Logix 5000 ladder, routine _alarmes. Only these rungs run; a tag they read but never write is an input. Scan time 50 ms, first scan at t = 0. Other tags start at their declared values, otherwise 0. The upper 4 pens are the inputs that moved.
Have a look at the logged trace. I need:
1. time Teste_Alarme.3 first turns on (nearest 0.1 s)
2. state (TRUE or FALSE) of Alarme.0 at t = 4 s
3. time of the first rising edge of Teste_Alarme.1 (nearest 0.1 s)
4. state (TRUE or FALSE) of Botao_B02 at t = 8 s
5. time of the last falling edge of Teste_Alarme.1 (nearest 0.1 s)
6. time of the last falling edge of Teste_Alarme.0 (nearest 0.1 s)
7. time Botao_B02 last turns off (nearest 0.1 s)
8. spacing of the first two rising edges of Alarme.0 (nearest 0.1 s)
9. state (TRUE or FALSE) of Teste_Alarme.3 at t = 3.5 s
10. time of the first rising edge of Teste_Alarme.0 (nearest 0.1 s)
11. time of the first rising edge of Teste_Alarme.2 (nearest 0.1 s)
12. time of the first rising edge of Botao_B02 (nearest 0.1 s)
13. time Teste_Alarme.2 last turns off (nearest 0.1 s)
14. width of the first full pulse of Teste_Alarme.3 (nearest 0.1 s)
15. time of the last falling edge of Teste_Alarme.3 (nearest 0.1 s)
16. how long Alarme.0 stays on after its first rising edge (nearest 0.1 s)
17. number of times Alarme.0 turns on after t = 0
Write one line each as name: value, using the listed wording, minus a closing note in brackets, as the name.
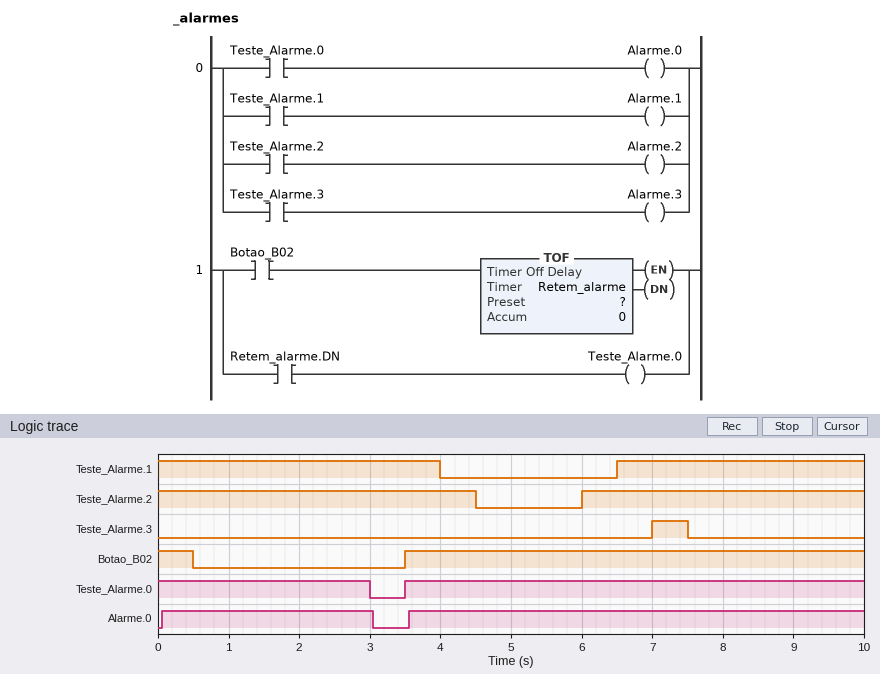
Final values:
time Teste_Alarme.3 first turns on: 7.0 s
state (TRUE or FALSE) of Alarme.0 at t = 4 s: TRUE
time of the first rising edge of Teste_Alarme.1: 6.5 s
state (TRUE or FALSE) of Botao_B02 at t = 8 s: TRUE
time of the last falling edge of Teste_Alarme.1: 4.0 s
time of the last falling edge of Teste_Alarme.0: 3.0 s
time Botao_B02 last turns off: 0.5 s
spacing of the first two rising edges of Alarme.0: 3.5 s
state (TRUE or FALSE) of Teste_Alarme.3 at t = 3.5 s: FALSE
time of the first rising edge of Teste_Alarme.0: 3.5 s
time of the first rising edge of Teste_Alarme.2: 6.0 s
time of the first rising edge of Botao_B02: 3.5 s
time Teste_Alarme.2 last turns off: 4.5 s
width of the first full pulse of Teste_Alarme.3: 0.5 s
time of the last falling edge of Teste_Alarme.3: 7.5 s
how long Alarme.0 stays on after its first rising edge: 3.0 s
number of times Alarme.0 turns on after t = 0: 2
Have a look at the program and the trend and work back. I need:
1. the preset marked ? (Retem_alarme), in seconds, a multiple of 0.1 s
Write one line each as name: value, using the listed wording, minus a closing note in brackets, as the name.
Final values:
the preset marked ? (Retem_alarme), in seconds, a multiple of 0.1 s: 2.5 s
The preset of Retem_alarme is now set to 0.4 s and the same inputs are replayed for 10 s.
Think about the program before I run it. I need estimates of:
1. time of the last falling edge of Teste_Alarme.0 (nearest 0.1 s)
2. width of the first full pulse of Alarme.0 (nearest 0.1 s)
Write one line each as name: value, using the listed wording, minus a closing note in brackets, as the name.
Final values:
time of the last falling edge of Teste_Alarme.0: 0.9 s
width of the first full pulse of Alarme.0: 0.9 s
